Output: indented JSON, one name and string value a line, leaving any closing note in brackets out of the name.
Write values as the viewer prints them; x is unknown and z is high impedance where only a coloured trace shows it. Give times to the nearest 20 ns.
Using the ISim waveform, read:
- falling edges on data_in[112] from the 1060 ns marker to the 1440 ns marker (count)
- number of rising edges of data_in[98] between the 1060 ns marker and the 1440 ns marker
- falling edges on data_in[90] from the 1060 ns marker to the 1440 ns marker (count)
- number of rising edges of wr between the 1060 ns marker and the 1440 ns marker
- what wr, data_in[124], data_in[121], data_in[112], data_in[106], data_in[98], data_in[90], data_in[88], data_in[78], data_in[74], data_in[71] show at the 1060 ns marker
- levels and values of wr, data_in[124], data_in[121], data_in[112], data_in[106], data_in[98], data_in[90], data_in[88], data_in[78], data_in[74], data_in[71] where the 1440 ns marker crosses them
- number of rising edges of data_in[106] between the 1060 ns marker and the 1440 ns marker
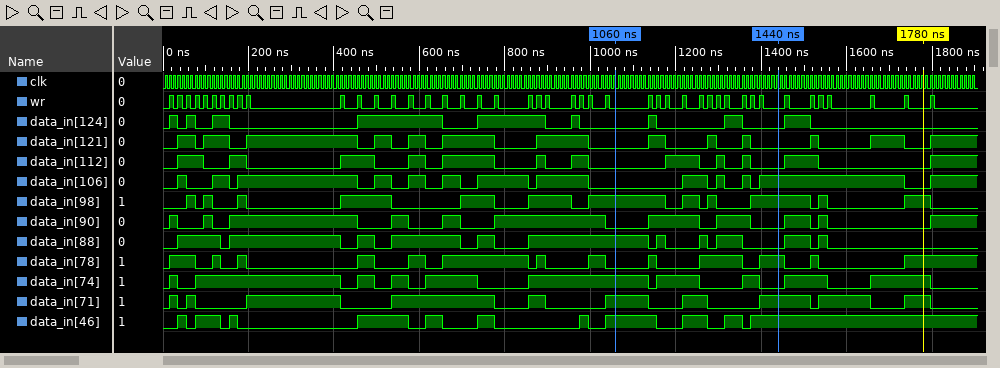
{
  "falling edges on data_in[112] from the 1060 ns marker to the 1440 ns marker": "3",
  "number of rising edges of data_in[98] between the 1060 ns marker and the 1440 ns marker": "3",
  "falling edges on data_in[90] from the 1060 ns marker to the 1440 ns marker": "2",
  "number of rising edges of wr between the 1060 ns marker and the 1440 ns marker": "11",
  "what wr, data_in[124], data_in[121], data_in[112], data_in[106], data_in[98], data_in[90], data_in[88], data_in[78], data_in[74], data_in[71] show at the 1060 ns marker": "wr=0, data_in[124]=0, data_in[121]=0, data_in[112]=0, data_in[106]=0, data_in[98]=1, data_in[90]=0, data_in[88]=1, data_in[78]=0, data_in[74]=1, data_in[71]=1",
  "levels and values of wr, data_in[124], data_in[121], data_in[112], data_in[106], data_in[98], data_in[90], data_in[88], data_in[78], data_in[74], data_in[71] where the 1440 ns marker crosses them": "wr=0, data_in[124]=0, data_in[121]=0, data_in[112]=0, data_in[106]=1, data_in[98]=1, data_in[90]=0, data_in[88]=0, data_in[78]=1, data_in[74]=0, data_in[71]=1",
  "number of rising edges of data_in[106] between the 1060 ns marker and the 1440 ns marker": "4"
}
